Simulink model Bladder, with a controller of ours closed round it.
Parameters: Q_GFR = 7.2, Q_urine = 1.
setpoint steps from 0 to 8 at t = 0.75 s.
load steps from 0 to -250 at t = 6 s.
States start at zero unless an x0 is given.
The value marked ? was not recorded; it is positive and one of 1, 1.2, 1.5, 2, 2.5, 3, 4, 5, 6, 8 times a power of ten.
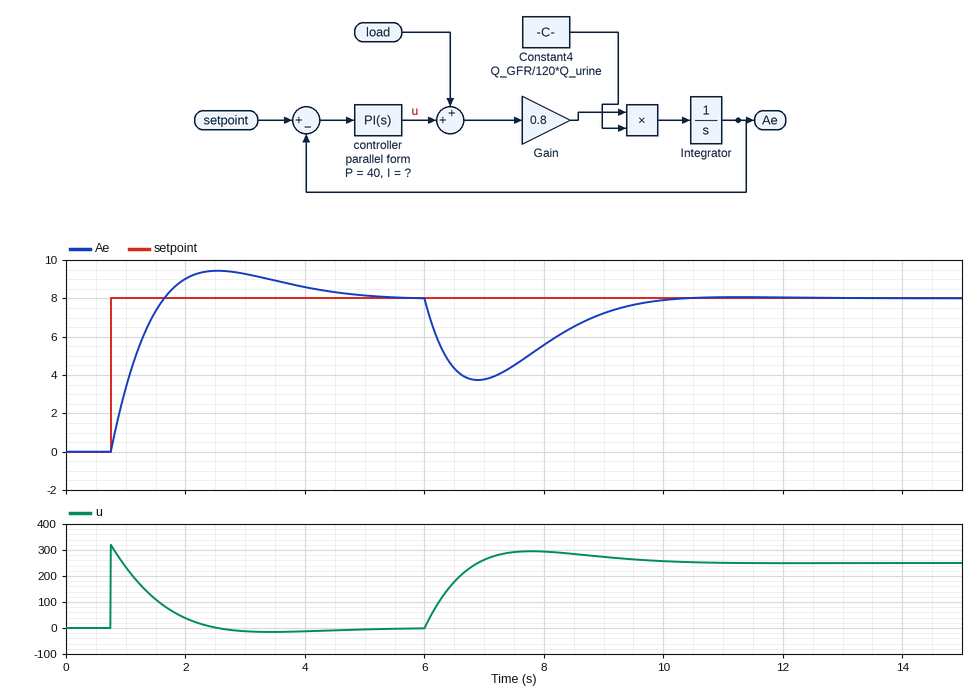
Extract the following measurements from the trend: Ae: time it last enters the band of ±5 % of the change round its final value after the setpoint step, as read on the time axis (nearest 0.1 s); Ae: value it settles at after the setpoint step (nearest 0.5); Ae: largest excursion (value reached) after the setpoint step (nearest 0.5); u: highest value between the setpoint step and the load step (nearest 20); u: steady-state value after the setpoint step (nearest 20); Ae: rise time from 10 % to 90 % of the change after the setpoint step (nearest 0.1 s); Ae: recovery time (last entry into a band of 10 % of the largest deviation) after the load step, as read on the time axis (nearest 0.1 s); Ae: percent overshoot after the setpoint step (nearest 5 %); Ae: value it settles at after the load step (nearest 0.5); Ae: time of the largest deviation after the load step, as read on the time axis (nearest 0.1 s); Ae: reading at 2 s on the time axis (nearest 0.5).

4.3 s
8.0
9.5
320
0
0.7 s
9.4 s
20 %
8.0
6.9 s
9.0
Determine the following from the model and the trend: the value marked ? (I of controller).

30
